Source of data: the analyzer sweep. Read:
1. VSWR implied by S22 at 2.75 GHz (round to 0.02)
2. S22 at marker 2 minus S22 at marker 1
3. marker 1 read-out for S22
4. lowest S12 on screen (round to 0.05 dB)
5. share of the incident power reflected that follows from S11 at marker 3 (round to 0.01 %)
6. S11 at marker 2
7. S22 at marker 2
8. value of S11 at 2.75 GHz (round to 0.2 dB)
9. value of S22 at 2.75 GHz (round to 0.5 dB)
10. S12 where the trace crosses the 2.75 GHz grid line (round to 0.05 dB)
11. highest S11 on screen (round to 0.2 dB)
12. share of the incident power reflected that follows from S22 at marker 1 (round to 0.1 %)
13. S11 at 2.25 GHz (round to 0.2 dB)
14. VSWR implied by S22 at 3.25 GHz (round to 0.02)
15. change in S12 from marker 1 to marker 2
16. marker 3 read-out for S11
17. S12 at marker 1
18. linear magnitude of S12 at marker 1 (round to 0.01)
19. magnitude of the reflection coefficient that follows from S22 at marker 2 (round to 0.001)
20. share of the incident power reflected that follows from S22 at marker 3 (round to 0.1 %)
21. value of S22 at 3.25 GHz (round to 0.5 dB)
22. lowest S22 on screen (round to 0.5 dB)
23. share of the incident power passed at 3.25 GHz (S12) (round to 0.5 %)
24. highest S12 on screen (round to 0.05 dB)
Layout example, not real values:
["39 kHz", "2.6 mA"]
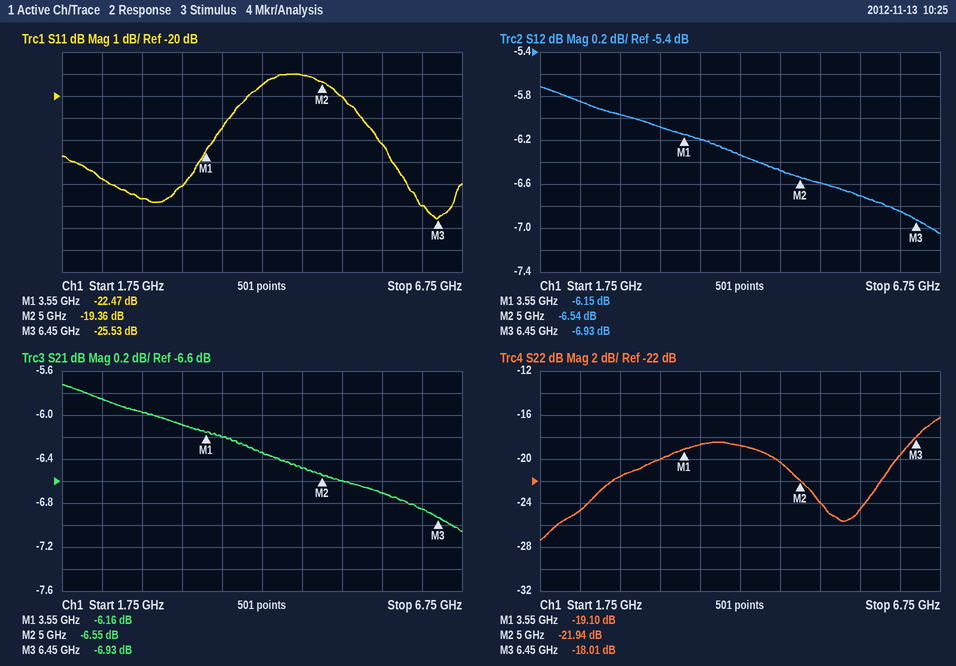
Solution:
["1.18", "-2.84 dB", "-19.10 dB", "-7.05 dB", "0.28 %", "-19.36 dB", "-21.94 dB", "-24.6 dB", "-21.5 dB", "-5.95 dB", "-19.0 dB", "1.2 %", "-23.8 dB", "1.22", "-0.39 dB", "-25.53 dB", "-6.15 dB", "0.49", "0.080", "1.6 %", "-20.0 dB", "-27.5 dB", "24.5 %", "-5.70 dB"]
